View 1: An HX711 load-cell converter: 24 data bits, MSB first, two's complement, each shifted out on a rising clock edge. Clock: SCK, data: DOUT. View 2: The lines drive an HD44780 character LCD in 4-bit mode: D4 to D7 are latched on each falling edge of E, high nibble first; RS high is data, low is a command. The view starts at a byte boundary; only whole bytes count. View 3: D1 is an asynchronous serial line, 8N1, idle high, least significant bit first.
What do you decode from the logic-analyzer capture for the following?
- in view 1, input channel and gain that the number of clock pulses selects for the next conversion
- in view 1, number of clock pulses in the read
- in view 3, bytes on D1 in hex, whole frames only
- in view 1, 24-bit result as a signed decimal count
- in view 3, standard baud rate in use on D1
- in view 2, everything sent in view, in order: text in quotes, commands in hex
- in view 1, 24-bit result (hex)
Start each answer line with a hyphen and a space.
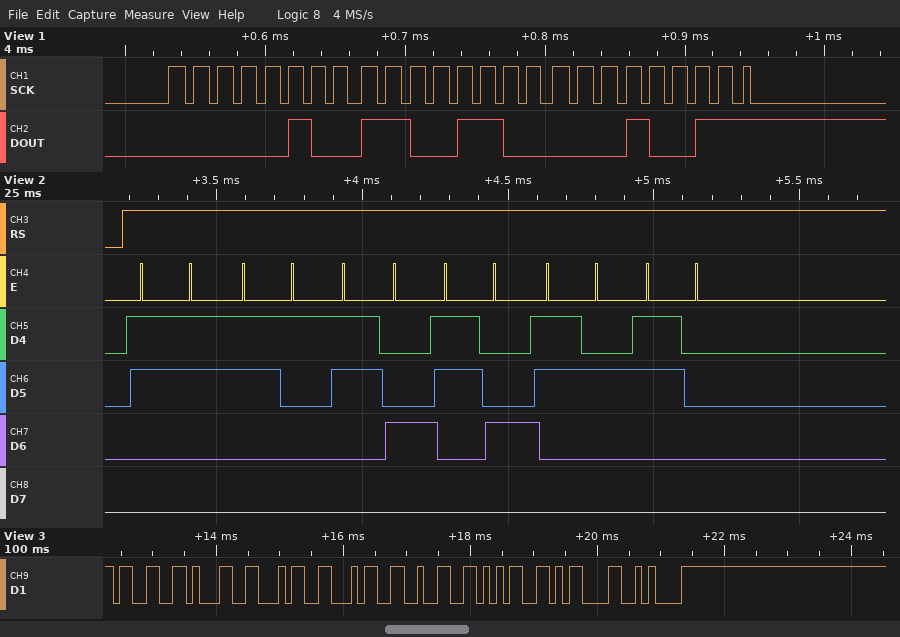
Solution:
- channel A, gain 128
- 25
- 33 31 34 34 32 35 0D 0A
- 314387
- 9600 baud
- "314420"
- 0x04CC13
